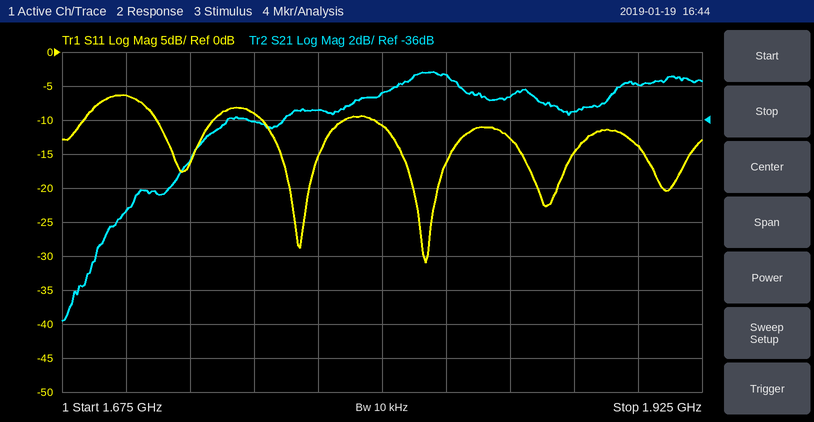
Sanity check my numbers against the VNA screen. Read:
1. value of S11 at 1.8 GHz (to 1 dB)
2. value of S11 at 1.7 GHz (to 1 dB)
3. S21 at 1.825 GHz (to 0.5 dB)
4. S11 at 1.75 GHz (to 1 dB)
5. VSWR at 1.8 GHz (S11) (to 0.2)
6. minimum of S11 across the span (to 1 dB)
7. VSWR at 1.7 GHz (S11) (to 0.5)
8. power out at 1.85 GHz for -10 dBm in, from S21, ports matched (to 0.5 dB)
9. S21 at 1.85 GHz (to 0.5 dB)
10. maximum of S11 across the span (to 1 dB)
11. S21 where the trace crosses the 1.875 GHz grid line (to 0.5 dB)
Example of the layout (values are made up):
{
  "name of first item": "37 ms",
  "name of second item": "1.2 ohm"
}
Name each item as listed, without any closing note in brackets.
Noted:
{
  "value of S11 at 1.8 GHz": "-11 dB",
  "value of S11 at 1.7 GHz": "-6 dB",
  "S21 at 1.825 GHz": "-33.5 dB",
  "S11 at 1.75 GHz": "-9 dB",
  "VSWR at 1.8 GHz (S11)": "1.8",
  "minimum of S11 across the span": "-31 dB",
  "VSWR at 1.7 GHz (S11)": "3.0",
  "power out at 1.85 GHz for -10 dBm in, from S21, ports matched": "-44.5 dBm",
  "S21 at 1.85 GHz": "-34.5 dB",
  "maximum of S11 across the span": "-6 dB",
  "S21 where the trace crosses the 1.875 GHz grid line": "-35.5 dB"
}
